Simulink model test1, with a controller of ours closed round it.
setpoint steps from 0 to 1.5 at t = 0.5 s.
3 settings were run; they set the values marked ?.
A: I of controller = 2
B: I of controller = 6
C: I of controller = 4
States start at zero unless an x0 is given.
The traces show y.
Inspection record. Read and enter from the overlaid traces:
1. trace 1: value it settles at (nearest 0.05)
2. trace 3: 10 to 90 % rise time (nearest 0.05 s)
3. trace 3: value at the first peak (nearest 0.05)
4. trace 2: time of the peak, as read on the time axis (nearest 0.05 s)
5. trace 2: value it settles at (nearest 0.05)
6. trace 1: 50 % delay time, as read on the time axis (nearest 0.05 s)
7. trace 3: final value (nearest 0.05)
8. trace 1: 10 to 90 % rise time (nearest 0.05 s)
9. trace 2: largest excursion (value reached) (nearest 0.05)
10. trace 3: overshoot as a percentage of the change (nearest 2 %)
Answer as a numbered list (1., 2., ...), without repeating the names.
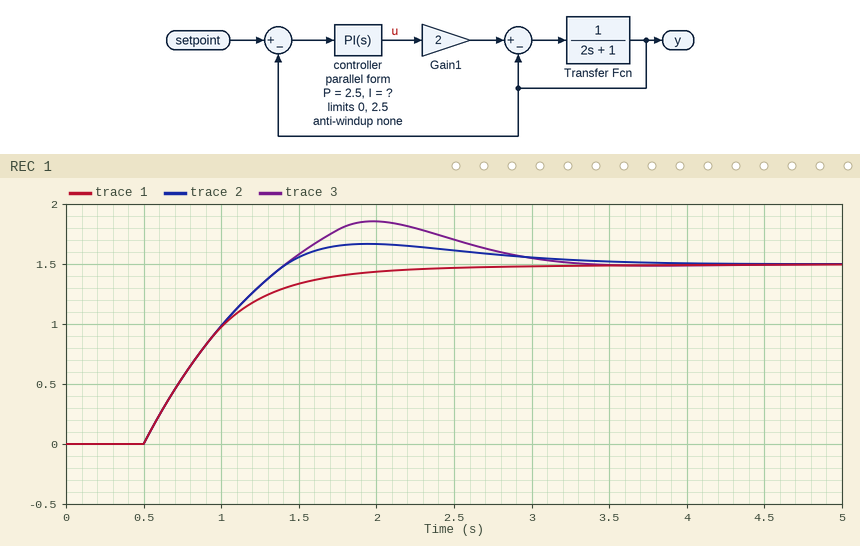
1. 1.50
2. 0.70 s
3. 1.85
4. 1.95 s
5. 1.50
6. 0.85 s
7. 1.50
8. 1.00 s
9. 1.65
10. 24 %
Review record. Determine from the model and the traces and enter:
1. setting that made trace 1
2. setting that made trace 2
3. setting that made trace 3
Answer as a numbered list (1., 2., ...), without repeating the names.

1. A
2. C
3. B
